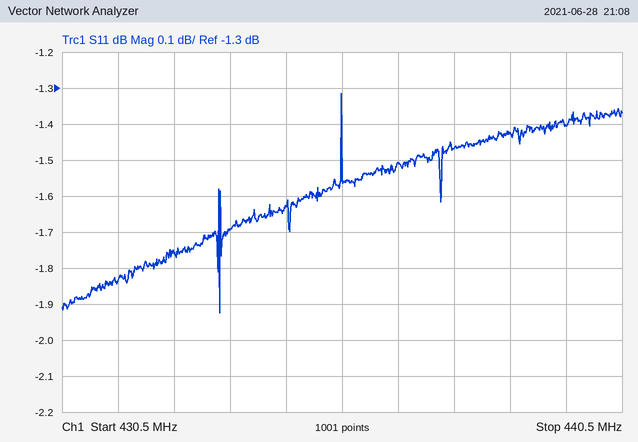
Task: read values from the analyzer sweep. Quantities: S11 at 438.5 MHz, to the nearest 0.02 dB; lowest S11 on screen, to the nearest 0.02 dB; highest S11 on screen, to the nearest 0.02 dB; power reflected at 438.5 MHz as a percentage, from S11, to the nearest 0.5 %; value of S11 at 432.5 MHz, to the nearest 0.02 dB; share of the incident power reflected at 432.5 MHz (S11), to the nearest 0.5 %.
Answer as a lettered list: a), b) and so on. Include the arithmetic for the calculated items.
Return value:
a) -1.42 dB
b) -1.92 dB
c) -1.32 dB
d) 10^(-1.42/10) ≈ 72.1 %, so 72.0 % to the nearest 0.5 %
e) -1.76 dB
f) 10^(-1.76/10) ≈ 66.7 %, so 66.5 % to the nearest 0.5 %
